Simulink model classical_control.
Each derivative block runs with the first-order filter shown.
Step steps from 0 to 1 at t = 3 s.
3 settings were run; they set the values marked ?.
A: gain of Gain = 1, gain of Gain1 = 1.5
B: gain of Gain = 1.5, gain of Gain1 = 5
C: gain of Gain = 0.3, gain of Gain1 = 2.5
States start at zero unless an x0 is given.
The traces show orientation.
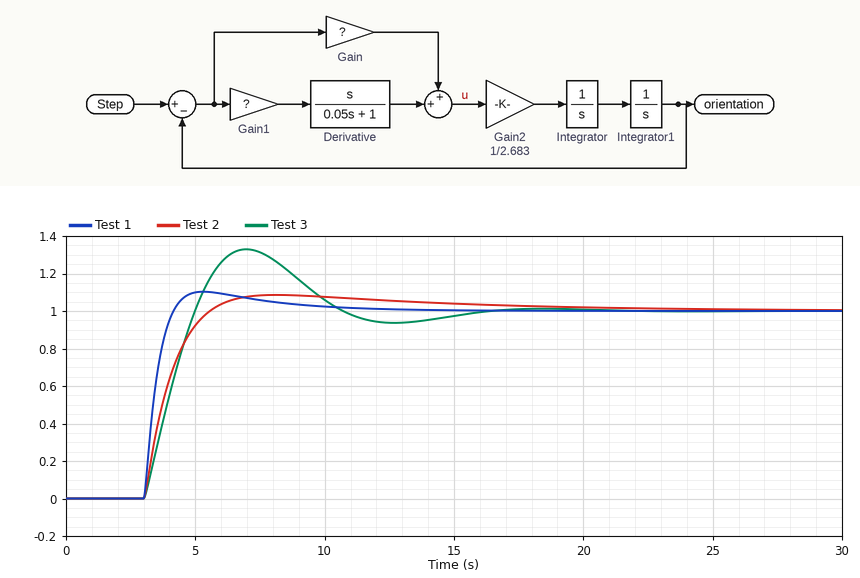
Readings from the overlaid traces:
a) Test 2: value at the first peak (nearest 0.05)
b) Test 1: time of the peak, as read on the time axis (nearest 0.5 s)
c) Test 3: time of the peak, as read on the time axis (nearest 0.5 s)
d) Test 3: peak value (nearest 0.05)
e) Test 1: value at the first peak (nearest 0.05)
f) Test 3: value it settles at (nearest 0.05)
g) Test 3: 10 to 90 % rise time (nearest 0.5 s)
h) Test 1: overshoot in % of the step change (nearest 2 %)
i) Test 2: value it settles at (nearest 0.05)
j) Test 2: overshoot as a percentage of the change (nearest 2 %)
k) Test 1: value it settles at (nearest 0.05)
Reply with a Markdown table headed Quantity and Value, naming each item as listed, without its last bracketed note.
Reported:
| Quantity | Value |
|---|---|
| Test 2: value at the first peak | 1.10 |
| Test 1: time of the peak, as read on the time axis | 5.5 s |
| Test 3: time of the peak, as read on the time axis | 7.0 s |
| Test 3: peak value | 1.35 |
| Test 1: value at the first peak | 1.10 |
| Test 3: value it settles at | 1.00 |
| Test 3: 10 to 90 % rise time | 1.5 s |
| Test 1: overshoot in % of the step change | 10 % |
| Test 2: value it settles at | 1.00 |
| Test 2: overshoot as a percentage of the change | 8 % |
| Test 1: value it settles at | 1.00 |
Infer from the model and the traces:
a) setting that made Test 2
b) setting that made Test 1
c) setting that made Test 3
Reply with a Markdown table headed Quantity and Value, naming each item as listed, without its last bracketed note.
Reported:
| Quantity | Value |
|---|---|
| setting that made Test 2 | C |
| setting that made Test 1 | B |
| setting that made Test 3 | A |
